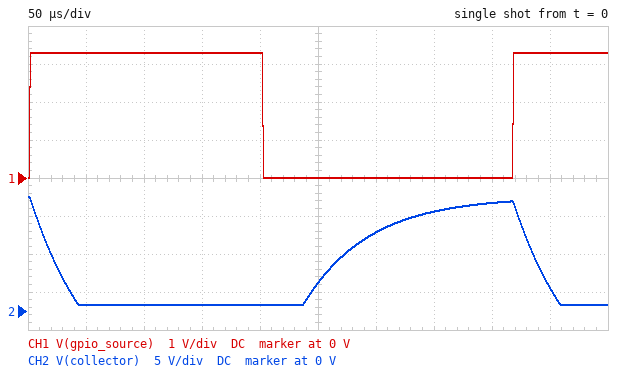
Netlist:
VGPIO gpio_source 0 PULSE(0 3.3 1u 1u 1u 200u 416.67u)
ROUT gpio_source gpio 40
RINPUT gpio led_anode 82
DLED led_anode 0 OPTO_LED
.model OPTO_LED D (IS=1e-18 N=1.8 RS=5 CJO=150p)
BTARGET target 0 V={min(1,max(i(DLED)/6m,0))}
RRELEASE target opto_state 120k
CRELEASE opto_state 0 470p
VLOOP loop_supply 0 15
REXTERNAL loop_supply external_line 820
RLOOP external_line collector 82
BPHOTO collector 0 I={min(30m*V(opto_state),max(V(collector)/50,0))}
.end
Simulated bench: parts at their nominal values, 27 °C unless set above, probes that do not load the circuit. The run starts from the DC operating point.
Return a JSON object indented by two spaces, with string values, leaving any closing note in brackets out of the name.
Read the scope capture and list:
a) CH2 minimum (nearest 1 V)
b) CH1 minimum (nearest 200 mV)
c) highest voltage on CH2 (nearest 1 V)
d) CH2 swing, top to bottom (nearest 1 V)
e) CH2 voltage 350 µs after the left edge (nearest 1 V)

{
  "CH2 minimum": "1 V",
  "CH1 minimum": "0 V",
  "highest voltage on CH2": "15 V",
  "CH2 swing, top to bottom": "14 V",
  "CH2 voltage 350 µs after the left edge": "13 V"
}
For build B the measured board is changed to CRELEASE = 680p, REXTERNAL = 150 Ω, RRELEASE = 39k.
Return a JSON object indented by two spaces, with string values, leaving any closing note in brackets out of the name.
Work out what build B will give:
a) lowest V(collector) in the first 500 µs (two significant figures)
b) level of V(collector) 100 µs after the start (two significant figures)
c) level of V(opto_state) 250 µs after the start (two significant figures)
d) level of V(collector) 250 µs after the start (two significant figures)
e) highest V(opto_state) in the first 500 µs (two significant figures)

{
  "lowest V(collector) in the first 500 µs": "8.0 V",
  "level of V(collector) 100 µs after the start": "8.2 V",
  "level of V(opto_state) 250 µs after the start": "170 mV",
  "level of V(collector) 250 µs after the start": "14 V",
  "highest V(opto_state) in the first 500 µs": "1.0 V"
}
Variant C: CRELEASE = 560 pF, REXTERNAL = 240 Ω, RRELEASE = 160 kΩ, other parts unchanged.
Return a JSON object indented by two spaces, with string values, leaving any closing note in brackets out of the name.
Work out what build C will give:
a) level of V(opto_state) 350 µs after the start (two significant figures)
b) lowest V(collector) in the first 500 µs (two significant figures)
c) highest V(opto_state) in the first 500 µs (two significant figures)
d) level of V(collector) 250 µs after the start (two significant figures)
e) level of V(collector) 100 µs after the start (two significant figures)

{
  "level of V(opto_state) 350 µs after the start": "170 mV",
  "lowest V(collector) in the first 500 µs": "6.4 V",
  "highest V(opto_state) in the first 500 µs": "890 mV",
  "level of V(collector) 250 µs after the start": "9.9 V",
  "level of V(collector) 100 µs after the start": "8.6 V"
}
